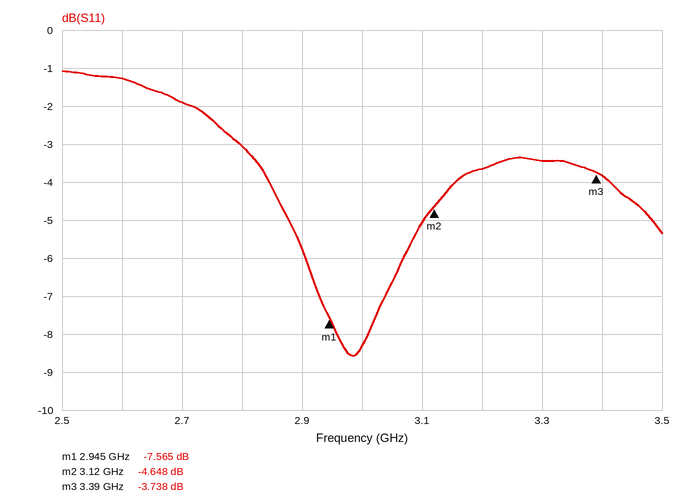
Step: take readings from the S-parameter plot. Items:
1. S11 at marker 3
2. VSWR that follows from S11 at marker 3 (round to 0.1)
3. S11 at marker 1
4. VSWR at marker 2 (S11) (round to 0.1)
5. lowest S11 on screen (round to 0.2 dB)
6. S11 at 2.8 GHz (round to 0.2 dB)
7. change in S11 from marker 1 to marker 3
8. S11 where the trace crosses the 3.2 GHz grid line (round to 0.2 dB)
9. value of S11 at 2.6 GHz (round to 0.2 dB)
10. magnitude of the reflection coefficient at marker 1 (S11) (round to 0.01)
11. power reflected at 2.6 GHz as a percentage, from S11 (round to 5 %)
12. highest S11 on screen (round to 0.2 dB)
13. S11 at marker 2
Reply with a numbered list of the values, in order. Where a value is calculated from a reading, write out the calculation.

1. -3.738 dB
2. (1 + 0.6503)/(1 − 0.6503) ≈ 4.7
3. -7.565 dB
4. (1 + 0.5856)/(1 − 0.5856) ≈ 3.8
5. -8.6 dB
6. -3.0 dB
7. -3.738 − (-7.565) = 3.827 dB
8. -3.6 dB
9. -1.2 dB
10. 10^(-7.565/20) ≈ 0.42
11. 10^(-1.2/10) ≈ 75.9 %, so 75 % to the nearest 5 %
12. -1.0 dB
13. -4.648 dB
